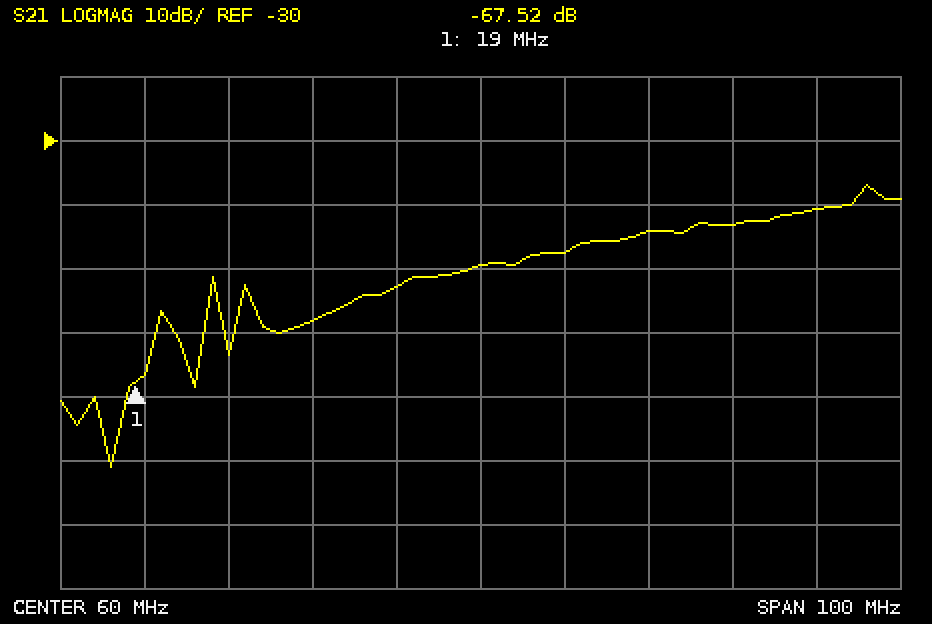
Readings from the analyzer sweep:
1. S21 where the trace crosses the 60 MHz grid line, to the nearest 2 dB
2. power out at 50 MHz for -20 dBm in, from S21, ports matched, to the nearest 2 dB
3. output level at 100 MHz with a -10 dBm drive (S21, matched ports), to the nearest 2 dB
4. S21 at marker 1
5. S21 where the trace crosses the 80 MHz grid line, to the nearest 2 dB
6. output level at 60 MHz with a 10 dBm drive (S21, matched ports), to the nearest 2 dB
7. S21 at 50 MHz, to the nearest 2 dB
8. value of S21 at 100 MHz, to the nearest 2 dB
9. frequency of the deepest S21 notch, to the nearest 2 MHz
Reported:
-50 dB
-72 dBm
-50 dBm
-67.52 dB
-44 dB
-40 dBm
-52 dB
-40 dB
16 MHz
